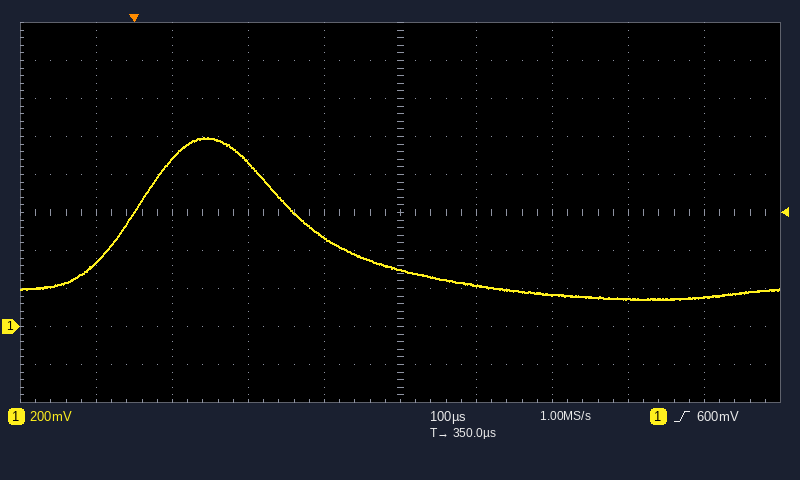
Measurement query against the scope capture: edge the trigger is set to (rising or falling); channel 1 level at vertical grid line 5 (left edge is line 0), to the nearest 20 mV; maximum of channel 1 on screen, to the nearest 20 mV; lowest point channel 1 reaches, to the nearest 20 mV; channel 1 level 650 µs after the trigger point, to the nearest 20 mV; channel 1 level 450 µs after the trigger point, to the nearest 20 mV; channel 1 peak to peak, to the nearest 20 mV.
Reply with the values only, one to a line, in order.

rising
300 mV
1.00 V
140 mV
140 mV
220 mV
860 mV
